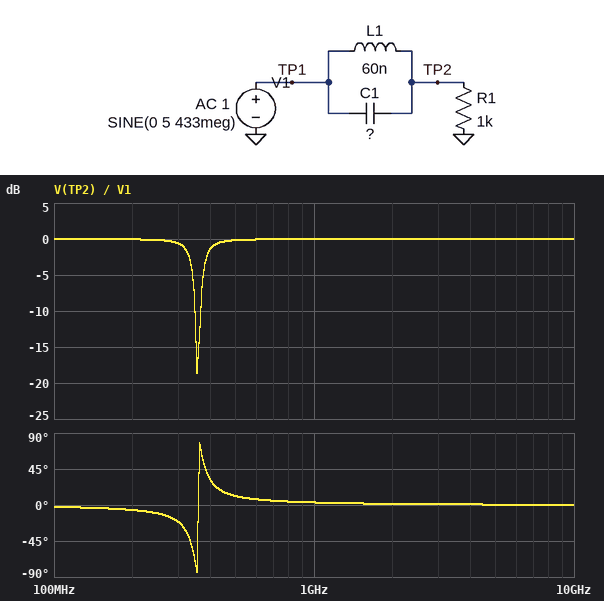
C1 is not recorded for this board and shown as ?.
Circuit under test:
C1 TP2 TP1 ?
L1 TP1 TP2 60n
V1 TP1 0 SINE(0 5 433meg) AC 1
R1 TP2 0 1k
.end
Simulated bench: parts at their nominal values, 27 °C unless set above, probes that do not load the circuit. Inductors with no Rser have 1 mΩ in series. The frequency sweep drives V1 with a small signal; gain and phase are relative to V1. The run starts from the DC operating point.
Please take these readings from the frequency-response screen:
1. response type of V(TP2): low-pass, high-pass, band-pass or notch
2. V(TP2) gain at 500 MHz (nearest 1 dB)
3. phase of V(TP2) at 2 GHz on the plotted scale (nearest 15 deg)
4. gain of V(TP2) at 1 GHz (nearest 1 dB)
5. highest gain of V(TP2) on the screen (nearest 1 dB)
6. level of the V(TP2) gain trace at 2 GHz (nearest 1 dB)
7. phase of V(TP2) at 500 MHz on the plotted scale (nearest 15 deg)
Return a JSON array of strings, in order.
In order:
["notch", "0 dB", "0 deg", "0 dB", "0 dB", "0 dB", "15 deg"]
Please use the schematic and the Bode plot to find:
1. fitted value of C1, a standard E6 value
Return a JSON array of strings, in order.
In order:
["3.3 pF"]
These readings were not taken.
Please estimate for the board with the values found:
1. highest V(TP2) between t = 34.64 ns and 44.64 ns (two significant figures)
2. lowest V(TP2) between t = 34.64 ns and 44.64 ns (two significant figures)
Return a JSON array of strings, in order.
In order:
["4.7 V", "-4.7 V"]
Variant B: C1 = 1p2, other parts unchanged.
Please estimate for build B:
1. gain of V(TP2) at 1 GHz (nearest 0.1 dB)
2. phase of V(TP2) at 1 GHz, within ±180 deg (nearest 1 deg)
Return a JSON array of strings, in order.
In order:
["-0.2 dB", "12 deg"]
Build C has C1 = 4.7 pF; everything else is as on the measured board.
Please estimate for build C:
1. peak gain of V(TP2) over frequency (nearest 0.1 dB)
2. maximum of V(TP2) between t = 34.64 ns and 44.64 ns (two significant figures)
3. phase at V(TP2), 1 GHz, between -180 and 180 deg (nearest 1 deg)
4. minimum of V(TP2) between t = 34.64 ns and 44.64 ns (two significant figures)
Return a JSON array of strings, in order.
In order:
["0 dB", "5.0 V", "2 deg", "-5.0 V"]
